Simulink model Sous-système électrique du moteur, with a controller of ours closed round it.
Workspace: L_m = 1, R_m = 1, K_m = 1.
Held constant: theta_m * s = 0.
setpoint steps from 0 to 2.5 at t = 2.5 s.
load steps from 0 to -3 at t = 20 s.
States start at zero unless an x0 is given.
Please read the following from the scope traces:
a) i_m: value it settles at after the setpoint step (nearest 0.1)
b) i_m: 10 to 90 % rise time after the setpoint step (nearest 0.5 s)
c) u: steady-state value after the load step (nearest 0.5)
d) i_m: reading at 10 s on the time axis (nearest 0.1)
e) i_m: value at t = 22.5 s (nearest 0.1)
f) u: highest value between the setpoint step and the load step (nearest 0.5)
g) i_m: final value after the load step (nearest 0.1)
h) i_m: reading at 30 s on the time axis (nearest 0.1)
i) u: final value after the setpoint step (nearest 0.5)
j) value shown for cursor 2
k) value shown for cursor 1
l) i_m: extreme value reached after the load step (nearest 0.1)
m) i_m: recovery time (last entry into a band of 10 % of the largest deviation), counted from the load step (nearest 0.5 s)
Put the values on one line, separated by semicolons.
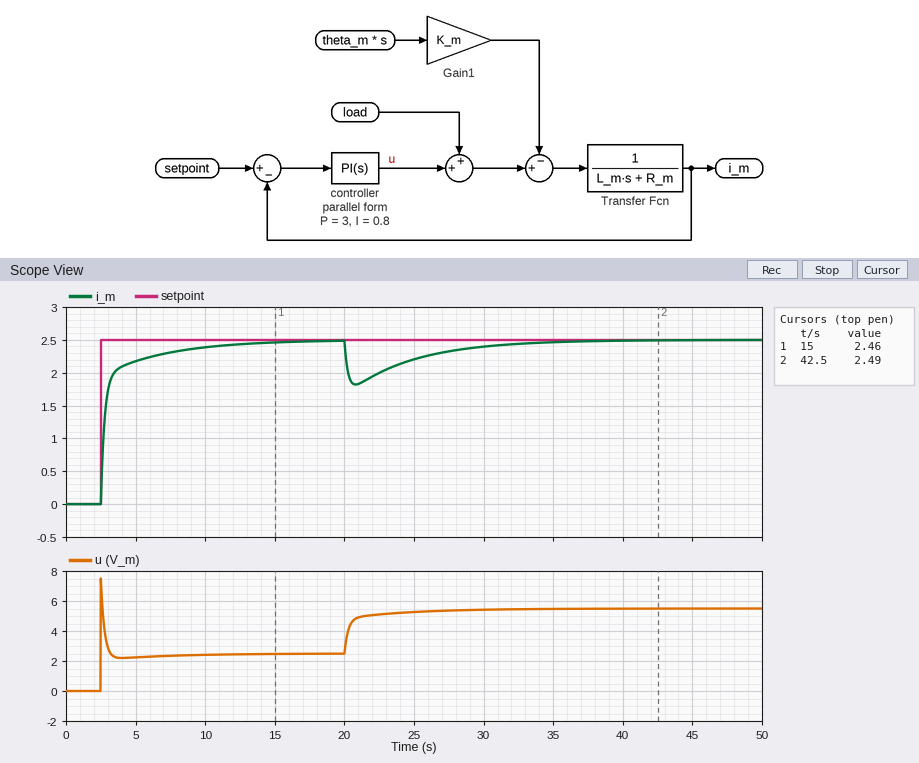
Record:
2.5; 3.5 s; 5.5; 2.4; 2.0; 7.5; 2.5; 2.4; 2.5; 2.49; 2.46; 1.8; 12.0 s
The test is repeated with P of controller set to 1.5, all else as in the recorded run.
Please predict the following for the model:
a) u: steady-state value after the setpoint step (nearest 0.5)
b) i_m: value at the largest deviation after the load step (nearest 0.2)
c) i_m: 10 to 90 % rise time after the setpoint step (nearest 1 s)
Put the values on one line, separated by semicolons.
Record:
2.5; 1.6; 3 s
